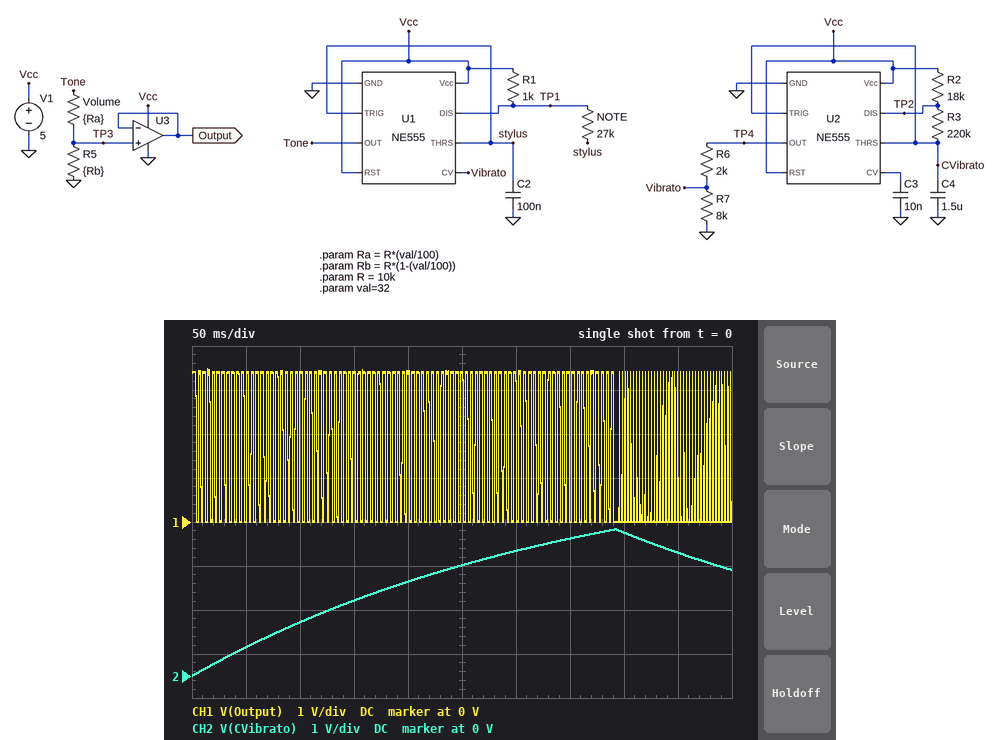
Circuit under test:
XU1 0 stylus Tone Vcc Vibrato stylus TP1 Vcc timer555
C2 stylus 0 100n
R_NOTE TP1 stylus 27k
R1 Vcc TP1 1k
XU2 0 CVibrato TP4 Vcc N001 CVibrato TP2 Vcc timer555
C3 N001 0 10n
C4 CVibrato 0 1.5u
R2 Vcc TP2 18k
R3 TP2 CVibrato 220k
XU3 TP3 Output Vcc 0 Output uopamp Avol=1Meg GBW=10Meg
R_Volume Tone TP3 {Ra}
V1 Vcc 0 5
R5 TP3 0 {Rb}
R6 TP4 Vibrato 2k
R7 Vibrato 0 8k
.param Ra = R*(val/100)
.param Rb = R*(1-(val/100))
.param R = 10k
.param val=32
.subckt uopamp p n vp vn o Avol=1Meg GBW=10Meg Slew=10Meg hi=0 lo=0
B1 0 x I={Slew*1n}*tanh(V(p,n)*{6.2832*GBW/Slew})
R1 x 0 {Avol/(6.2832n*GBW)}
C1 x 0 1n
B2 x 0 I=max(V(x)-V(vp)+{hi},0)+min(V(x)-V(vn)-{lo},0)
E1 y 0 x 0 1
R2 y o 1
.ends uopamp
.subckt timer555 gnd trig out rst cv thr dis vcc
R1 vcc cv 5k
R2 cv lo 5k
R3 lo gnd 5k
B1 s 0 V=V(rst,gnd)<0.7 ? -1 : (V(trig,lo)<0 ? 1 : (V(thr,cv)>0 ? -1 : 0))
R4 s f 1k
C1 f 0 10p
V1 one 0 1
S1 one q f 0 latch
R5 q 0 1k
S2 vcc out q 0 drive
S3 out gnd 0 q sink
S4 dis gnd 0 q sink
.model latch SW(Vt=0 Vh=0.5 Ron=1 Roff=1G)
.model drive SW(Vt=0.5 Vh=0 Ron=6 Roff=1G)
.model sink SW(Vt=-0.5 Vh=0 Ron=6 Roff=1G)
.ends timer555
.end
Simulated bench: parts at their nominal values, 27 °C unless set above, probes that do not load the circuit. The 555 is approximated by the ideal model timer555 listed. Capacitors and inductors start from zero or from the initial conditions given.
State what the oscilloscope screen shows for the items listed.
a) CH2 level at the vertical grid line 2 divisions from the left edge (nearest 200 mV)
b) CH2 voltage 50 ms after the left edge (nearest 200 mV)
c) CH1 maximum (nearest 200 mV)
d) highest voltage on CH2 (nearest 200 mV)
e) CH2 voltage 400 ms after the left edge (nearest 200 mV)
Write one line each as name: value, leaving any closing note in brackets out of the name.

CH2 level at the vertical grid line 2 divisions from the left edge: 1.2 V
CH2 voltage 50 ms after the left edge: 600 mV
CH1 maximum: 3.4 V
highest voltage on CH2: 3.4 V
CH2 voltage 400 ms after the left edge: 3.2 V
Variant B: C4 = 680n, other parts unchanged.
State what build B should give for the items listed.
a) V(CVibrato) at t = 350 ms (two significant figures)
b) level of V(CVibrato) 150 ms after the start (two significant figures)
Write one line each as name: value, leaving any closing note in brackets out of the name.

V(CVibrato) at t = 350 ms: 2.8 V
level of V(CVibrato) 150 ms after the start: 3.0 V
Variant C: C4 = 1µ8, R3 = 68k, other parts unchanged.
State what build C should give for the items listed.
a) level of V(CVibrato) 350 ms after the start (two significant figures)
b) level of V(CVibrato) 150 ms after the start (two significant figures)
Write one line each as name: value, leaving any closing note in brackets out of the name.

level of V(CVibrato) 350 ms after the start: 3.2 V
level of V(CVibrato) 150 ms after the start: 3.1 V
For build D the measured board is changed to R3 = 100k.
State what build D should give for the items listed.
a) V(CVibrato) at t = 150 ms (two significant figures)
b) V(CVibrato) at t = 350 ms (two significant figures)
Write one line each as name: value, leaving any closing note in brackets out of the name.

V(CVibrato) at t = 150 ms: 2.9 V
V(CVibrato) at t = 350 ms: 2.5 V
